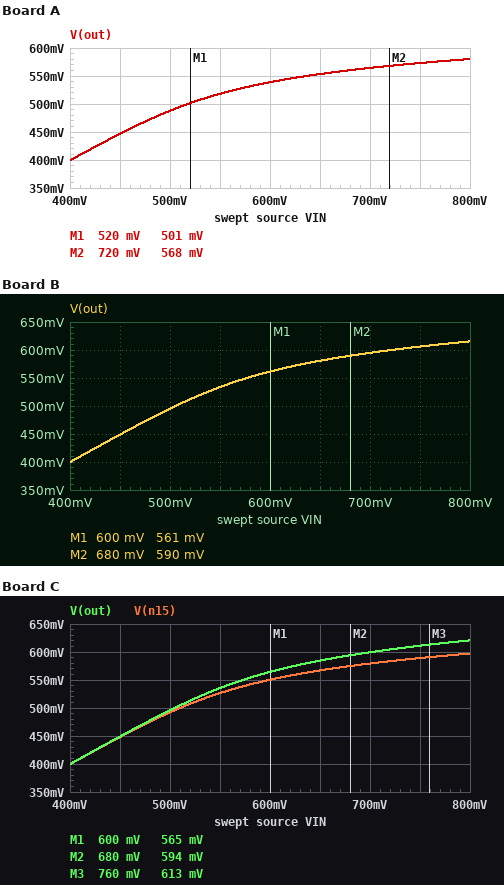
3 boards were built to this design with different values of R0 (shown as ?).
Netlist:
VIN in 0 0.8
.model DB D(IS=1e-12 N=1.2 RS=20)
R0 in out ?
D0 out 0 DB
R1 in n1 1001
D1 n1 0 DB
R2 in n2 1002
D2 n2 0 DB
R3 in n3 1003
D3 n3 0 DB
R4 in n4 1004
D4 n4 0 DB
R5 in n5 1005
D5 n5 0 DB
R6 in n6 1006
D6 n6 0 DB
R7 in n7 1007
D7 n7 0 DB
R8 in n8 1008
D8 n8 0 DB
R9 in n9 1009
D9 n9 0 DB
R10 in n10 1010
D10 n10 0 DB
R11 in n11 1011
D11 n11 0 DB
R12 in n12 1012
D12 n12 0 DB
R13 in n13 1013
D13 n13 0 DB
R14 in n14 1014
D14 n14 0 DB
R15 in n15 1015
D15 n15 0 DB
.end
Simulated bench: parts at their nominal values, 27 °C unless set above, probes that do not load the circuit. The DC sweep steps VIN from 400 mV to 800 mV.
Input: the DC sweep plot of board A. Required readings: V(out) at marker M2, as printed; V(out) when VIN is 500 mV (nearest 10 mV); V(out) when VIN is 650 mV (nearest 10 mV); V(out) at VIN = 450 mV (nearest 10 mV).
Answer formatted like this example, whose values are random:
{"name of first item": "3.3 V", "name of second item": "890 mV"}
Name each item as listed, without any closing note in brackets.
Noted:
{"V(out) at marker M2, as printed": "568 mV", "V(out) when VIN is 500 mV": "490 mV", "V(out) when VIN is 650 mV": "550 mV", "V(out) at VIN = 450 mV": "450 mV"}
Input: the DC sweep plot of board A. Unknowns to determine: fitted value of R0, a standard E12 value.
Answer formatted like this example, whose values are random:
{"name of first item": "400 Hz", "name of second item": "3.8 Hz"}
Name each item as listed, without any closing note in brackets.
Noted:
{"fitted value of R0, a standard E12 value": "1.8 kΩ"}
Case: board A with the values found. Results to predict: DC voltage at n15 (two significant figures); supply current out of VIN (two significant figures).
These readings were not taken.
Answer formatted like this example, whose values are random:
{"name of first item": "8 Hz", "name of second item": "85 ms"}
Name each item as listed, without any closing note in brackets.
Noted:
{"DC voltage at n15": "600 mV", "supply current out of VIN": "3.1 mA"}
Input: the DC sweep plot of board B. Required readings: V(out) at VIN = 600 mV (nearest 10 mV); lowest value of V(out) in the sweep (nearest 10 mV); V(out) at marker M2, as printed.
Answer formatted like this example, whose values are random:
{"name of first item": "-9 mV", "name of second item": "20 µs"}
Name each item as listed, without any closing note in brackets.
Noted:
{"V(out) at VIN = 600 mV": "560 mV", "lowest value of V(out) in the sweep": "400 mV", "V(out) at marker M2, as printed": "590 mV"}
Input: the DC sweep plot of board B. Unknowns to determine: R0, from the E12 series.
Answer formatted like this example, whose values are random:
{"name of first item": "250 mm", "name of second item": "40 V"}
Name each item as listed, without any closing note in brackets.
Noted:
{"R0, from the E12 series": "560 Ω"}
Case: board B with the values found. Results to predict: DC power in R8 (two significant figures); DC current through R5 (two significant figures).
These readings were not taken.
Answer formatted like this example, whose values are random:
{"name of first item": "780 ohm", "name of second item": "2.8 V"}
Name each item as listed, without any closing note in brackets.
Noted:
{"DC power in R8": "41 µW", "DC current through R5": "200 µA"}
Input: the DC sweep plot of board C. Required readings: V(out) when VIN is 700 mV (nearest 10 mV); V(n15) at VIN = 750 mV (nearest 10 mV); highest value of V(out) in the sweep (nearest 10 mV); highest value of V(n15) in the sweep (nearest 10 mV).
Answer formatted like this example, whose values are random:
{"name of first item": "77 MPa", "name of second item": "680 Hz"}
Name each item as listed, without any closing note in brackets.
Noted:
{"V(out) when VIN is 700 mV": "600 mV", "V(n15) at VIN = 750 mV": "590 mV", "highest value of V(out) in the sweep": "620 mV", "highest value of V(n15) in the sweep": "600 mV"}
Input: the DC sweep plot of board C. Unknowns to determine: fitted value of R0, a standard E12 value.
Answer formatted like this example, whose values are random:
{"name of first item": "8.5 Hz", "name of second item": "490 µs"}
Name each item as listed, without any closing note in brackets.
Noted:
{"fitted value of R0, a standard E12 value": "470 Ω"}
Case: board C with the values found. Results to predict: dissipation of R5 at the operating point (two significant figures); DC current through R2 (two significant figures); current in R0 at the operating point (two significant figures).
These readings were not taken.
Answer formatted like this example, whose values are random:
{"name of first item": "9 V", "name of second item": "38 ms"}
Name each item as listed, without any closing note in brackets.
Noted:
{"dissipation of R5 at the operating point": "41 µW", "DC current through R2": "200 µA", "current in R0 at the operating point": "380 µA"}
